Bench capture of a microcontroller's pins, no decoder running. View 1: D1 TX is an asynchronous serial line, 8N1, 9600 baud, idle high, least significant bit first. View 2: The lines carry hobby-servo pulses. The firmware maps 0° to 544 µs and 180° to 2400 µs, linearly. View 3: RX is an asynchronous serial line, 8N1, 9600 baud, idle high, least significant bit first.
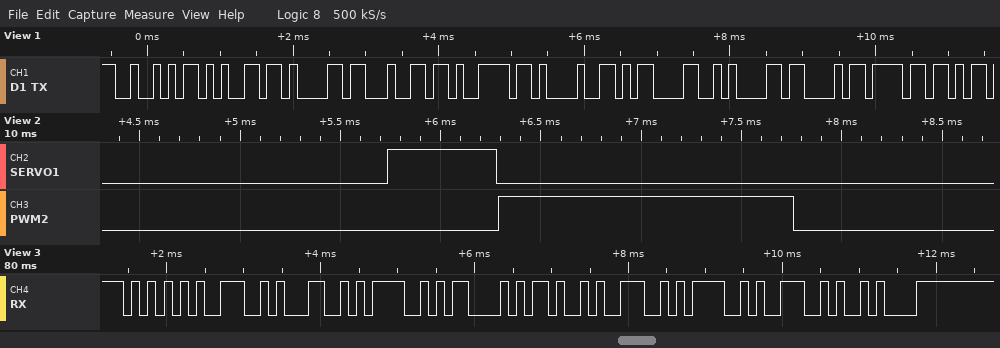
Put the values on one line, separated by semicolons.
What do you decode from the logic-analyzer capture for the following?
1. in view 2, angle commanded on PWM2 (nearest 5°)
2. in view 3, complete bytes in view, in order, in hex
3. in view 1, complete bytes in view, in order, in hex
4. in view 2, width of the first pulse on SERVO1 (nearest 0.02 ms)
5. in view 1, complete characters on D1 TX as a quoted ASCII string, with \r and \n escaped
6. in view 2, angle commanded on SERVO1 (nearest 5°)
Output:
90°; 0x55 0x4E 0x4C 0x4F 0x43 0x4B 0x4E 0x4F 0x4E 0x0A; 52 65 61 64 79 21 0D 0A 43 6F; 0.54 ms; "Ready!\r\nCo"; 0°
